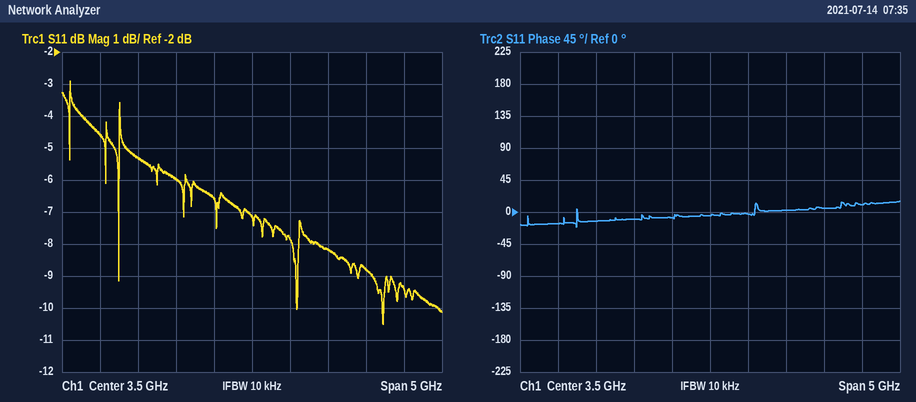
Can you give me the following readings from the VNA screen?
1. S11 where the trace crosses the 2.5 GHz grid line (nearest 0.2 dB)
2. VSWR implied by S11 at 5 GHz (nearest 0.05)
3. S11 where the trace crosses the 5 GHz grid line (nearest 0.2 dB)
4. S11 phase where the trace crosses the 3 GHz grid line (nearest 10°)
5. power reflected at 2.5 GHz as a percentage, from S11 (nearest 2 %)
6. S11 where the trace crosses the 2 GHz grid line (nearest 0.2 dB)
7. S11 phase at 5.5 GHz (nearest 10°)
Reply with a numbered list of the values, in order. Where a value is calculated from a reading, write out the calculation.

1. -6.0 dB
2. |Γ| = 10^(-8.8/20) = 0.3631; VSWR = (1 + 0.3631)/(1 − 0.3631) ≈ 2.14, so 2.15 to the nearest 0.05
3. -8.8 dB
4. -10°
5. 10^(-6/10) ≈ 25.1 %, so 26 % to the nearest 2 %
6. -5.4 dB
7. 10°
